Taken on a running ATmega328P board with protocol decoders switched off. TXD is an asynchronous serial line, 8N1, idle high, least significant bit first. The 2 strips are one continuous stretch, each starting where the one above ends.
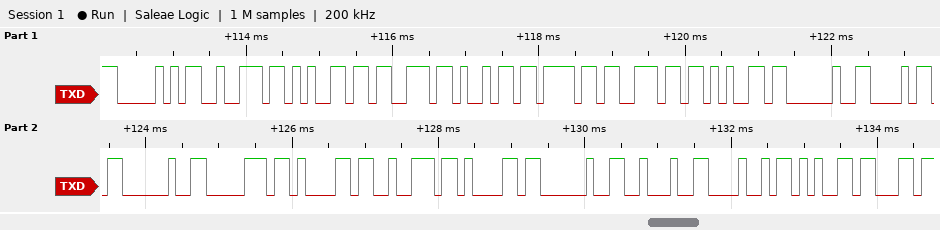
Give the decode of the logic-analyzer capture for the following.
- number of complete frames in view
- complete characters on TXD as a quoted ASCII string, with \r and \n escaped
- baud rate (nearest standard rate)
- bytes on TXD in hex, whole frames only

19
"Presione h para \"He"
9600 baud
0x50 0x72 0x65 0x73 0x69 0x6F 0x6E 0x65 0x20 0x68 0x20 0x70 0x61 0x72 0x61 0x20 0x22 0x48 0x65
